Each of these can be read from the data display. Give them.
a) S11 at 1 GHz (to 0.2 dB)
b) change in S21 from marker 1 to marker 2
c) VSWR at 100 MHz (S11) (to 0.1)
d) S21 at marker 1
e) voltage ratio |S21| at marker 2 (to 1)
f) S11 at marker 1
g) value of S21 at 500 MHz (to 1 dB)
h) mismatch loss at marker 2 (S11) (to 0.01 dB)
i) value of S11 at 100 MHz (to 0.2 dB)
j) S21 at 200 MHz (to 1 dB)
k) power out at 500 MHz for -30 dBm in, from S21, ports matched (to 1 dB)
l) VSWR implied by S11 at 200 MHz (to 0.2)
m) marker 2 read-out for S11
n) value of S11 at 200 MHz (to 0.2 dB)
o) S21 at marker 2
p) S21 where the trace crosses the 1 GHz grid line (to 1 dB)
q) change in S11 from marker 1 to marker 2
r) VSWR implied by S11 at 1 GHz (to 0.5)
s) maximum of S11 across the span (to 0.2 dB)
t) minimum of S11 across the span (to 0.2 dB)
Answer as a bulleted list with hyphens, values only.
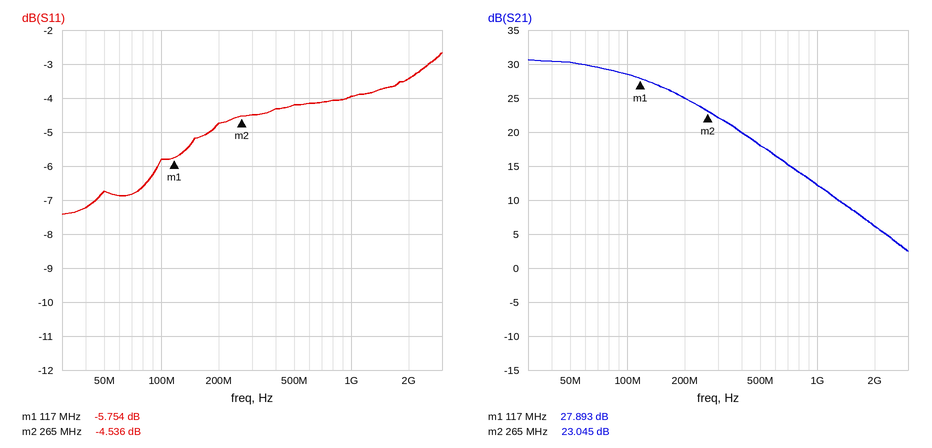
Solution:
- -4.0 dB
- -4.848 dB
- 3.1
- 27.893 dB
- 14
- -5.754 dB
- 18 dB
- 1.88 dB
- -5.8 dB
- 25 dB
- -12 dBm
- 3.8
- -4.536 dB
- -4.8 dB
- 23.045 dB
- 12 dB
- 1.218 dB
- 4.5
- -2.6 dB
- -7.4 dB
